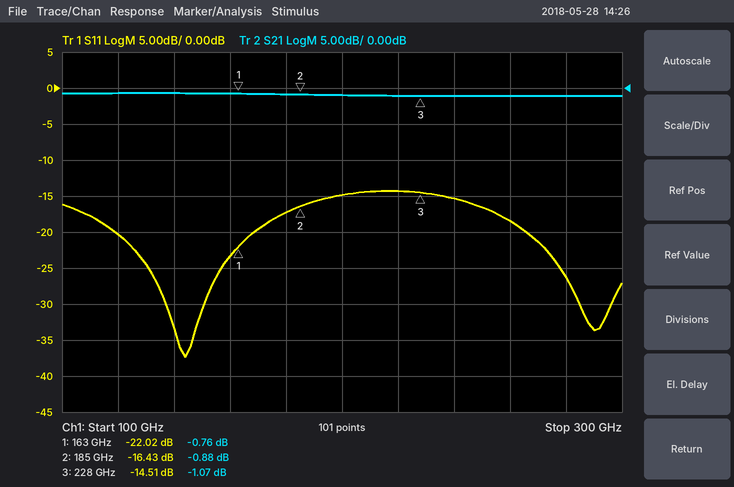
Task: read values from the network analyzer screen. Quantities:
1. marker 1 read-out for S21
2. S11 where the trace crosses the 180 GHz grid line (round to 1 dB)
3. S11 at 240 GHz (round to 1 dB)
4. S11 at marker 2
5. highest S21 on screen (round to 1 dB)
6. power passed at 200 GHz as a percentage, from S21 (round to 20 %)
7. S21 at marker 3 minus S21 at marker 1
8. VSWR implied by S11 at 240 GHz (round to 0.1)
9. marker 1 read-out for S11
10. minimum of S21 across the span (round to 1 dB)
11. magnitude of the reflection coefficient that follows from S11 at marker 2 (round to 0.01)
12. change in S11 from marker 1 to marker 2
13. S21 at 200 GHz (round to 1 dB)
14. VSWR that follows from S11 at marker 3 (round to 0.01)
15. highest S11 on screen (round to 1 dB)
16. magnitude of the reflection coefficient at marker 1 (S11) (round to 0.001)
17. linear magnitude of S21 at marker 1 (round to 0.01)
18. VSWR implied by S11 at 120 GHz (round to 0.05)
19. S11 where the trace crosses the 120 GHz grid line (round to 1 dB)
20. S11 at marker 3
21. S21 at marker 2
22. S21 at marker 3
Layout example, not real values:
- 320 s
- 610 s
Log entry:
- -0.76 dB
- -17 dB
- -15 dB
- -16.43 dB
- -1 dB
- 80 %
- -0.31 dB
- 1.4
- -22.02 dB
- -1 dB
- 0.15
- 5.59 dB
- -1 dB
- 1.46
- -14 dB
- 0.079
- 0.92
- 1.20
- -20 dB
- -14.51 dB
- -0.88 dB
- -1.07 dB
